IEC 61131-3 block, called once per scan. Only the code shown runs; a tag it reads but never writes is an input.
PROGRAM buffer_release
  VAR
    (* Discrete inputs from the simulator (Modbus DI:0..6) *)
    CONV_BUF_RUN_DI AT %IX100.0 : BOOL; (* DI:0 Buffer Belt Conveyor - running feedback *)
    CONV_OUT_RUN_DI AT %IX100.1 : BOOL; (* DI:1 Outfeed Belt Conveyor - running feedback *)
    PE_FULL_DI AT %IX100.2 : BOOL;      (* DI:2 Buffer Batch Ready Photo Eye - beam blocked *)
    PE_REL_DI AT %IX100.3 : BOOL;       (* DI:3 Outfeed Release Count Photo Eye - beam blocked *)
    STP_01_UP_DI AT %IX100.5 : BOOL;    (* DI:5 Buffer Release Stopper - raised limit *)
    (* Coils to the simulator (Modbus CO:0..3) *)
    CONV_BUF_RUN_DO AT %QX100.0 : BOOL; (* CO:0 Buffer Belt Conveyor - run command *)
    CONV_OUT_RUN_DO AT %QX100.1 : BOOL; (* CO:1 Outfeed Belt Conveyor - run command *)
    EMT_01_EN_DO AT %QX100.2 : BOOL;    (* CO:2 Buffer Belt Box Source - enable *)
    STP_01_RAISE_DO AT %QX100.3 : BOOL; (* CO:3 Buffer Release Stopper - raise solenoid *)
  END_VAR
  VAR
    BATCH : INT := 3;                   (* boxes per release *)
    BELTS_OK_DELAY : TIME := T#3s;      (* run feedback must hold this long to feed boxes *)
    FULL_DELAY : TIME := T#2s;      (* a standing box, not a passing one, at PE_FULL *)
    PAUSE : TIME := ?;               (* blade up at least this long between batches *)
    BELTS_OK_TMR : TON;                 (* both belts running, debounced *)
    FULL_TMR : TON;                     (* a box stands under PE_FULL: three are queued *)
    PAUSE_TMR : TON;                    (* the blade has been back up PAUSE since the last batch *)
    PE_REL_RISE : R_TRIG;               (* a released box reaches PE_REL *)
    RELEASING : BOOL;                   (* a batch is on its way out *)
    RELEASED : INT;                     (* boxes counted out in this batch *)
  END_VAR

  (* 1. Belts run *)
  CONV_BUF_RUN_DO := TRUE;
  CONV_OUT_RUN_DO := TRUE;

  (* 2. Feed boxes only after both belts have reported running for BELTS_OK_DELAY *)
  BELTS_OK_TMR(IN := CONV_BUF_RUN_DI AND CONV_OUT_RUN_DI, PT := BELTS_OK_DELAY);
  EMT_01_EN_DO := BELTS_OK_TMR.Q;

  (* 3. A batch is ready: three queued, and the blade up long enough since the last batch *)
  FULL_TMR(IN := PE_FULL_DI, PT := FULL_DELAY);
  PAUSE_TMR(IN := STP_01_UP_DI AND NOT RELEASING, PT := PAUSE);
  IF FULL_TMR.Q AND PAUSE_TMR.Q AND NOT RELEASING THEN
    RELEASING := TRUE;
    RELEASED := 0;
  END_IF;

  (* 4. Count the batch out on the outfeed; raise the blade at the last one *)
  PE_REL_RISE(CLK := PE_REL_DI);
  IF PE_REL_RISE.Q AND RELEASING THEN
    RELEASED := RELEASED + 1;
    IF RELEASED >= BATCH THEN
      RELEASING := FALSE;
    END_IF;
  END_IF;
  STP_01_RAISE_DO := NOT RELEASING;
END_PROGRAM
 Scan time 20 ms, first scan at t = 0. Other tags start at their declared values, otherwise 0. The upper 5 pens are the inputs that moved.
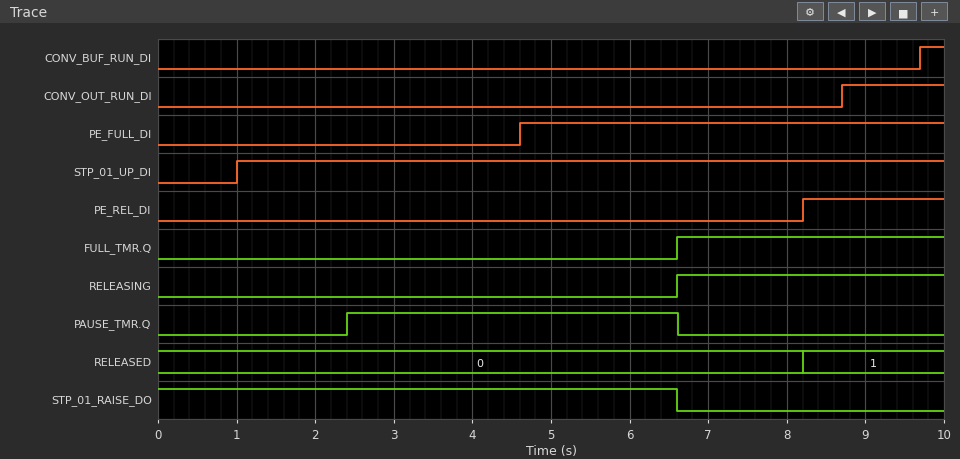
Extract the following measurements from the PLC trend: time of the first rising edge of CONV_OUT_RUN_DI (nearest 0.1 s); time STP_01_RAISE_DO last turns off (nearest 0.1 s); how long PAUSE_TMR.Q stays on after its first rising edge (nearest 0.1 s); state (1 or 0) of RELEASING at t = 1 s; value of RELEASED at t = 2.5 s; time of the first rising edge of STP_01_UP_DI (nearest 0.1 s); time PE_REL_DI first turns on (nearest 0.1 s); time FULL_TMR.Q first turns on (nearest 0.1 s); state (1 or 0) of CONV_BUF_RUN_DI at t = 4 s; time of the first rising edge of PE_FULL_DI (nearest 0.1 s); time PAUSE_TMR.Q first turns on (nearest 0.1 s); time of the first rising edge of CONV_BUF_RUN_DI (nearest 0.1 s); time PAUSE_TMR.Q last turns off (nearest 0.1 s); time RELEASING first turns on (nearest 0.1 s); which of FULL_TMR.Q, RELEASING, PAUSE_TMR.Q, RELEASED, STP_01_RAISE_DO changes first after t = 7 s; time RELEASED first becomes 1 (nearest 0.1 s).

8.7 s
6.6 s
4.2 s
0
0
1.0 s
8.2 s
6.6 s
0
4.6 s
2.4 s
9.7 s
6.6 s
6.6 s
RELEASED
8.2 s
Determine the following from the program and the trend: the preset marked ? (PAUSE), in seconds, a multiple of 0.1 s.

1.4 s
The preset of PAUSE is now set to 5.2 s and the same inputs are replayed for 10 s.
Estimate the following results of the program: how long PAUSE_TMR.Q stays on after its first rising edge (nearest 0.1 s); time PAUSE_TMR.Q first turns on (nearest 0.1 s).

0.4 s
6.2 s
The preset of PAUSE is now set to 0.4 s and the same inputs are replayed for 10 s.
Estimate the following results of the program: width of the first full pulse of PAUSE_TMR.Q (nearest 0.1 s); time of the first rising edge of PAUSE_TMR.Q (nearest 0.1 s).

5.2 s
1.4 s
